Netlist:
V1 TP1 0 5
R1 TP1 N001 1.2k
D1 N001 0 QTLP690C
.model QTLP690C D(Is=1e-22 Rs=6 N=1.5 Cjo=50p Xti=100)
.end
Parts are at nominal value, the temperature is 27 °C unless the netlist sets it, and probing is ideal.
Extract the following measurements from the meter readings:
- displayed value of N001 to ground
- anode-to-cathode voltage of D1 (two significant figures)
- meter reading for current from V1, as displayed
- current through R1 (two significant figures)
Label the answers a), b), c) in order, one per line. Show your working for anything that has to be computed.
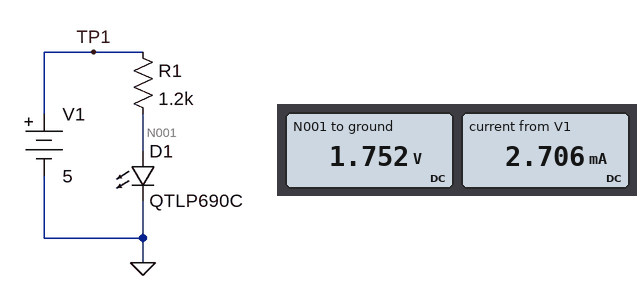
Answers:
a) 1.752 V
b) 1.752 V = 1.8 V
c) 2.706 mA
d) (5 V - 1.752 V) / 1.2 kΩ = 2.7 mA
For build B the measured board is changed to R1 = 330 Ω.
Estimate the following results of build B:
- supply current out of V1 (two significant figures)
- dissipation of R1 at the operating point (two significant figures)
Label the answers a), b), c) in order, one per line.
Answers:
a) 9.6 mA
b) 30 mW
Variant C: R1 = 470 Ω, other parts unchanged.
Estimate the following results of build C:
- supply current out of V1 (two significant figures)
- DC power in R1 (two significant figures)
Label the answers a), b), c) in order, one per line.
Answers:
a) 6.8 mA
b) 22 mW
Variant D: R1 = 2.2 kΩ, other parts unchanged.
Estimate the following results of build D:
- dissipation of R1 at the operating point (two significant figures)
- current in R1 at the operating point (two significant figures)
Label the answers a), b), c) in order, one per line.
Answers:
a) 4.9 mW
b) 1.5 mA
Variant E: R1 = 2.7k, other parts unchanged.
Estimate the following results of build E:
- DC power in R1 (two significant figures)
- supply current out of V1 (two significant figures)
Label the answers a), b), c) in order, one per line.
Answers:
a) 4.0 mW
b) 1.2 mA
